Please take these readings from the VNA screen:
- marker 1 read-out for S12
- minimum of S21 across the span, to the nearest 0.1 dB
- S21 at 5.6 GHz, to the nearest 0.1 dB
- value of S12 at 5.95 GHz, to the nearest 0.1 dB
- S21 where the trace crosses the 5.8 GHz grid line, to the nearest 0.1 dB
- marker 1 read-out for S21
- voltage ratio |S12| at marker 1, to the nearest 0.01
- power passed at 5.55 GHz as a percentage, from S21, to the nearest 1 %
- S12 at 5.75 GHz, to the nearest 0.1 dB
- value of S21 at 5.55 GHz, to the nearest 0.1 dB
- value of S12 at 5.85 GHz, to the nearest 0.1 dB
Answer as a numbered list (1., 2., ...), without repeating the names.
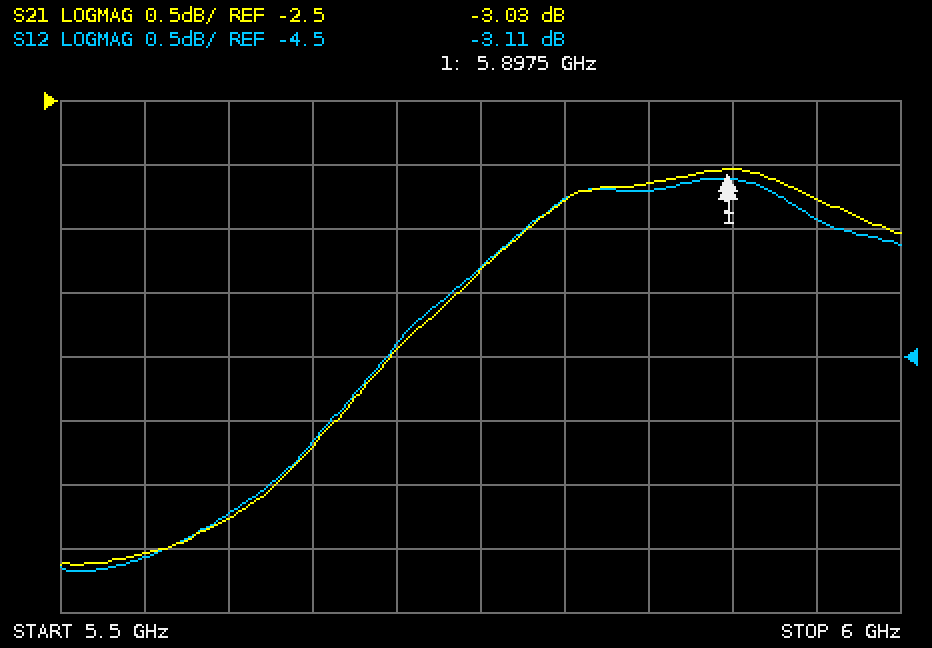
1. -3.11 dB
2. -6.1 dB
3. -5.8 dB
4. -3.4 dB
5. -3.3 dB
6. -3.03 dB
7. 0.70
8. 25 %
9. -3.8 dB
10. -6.0 dB
11. -3.2 dB
